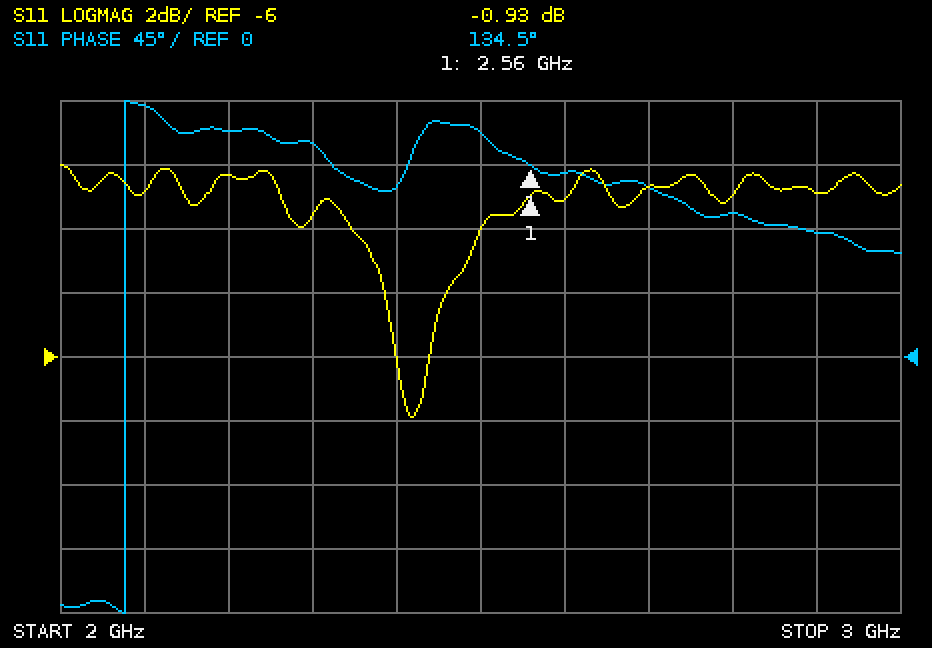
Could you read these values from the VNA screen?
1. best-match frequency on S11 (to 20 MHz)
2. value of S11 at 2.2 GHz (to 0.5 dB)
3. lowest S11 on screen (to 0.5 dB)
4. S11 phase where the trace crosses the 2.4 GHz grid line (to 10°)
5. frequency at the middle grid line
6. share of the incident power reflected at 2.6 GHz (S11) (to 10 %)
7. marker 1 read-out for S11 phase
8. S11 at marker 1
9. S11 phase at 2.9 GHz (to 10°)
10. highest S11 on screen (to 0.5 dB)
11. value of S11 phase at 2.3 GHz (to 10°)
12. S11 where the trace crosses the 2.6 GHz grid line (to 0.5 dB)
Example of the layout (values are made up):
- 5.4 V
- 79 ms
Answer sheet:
- 2.42 GHz
- -0.5 dB
- -8.0 dB
- 120°
- 2.5 GHz
- 80 %
- 134.5°
- -0.93 dB
- 90°
- 0.0 dB
- 150°
- -1.0 dB
